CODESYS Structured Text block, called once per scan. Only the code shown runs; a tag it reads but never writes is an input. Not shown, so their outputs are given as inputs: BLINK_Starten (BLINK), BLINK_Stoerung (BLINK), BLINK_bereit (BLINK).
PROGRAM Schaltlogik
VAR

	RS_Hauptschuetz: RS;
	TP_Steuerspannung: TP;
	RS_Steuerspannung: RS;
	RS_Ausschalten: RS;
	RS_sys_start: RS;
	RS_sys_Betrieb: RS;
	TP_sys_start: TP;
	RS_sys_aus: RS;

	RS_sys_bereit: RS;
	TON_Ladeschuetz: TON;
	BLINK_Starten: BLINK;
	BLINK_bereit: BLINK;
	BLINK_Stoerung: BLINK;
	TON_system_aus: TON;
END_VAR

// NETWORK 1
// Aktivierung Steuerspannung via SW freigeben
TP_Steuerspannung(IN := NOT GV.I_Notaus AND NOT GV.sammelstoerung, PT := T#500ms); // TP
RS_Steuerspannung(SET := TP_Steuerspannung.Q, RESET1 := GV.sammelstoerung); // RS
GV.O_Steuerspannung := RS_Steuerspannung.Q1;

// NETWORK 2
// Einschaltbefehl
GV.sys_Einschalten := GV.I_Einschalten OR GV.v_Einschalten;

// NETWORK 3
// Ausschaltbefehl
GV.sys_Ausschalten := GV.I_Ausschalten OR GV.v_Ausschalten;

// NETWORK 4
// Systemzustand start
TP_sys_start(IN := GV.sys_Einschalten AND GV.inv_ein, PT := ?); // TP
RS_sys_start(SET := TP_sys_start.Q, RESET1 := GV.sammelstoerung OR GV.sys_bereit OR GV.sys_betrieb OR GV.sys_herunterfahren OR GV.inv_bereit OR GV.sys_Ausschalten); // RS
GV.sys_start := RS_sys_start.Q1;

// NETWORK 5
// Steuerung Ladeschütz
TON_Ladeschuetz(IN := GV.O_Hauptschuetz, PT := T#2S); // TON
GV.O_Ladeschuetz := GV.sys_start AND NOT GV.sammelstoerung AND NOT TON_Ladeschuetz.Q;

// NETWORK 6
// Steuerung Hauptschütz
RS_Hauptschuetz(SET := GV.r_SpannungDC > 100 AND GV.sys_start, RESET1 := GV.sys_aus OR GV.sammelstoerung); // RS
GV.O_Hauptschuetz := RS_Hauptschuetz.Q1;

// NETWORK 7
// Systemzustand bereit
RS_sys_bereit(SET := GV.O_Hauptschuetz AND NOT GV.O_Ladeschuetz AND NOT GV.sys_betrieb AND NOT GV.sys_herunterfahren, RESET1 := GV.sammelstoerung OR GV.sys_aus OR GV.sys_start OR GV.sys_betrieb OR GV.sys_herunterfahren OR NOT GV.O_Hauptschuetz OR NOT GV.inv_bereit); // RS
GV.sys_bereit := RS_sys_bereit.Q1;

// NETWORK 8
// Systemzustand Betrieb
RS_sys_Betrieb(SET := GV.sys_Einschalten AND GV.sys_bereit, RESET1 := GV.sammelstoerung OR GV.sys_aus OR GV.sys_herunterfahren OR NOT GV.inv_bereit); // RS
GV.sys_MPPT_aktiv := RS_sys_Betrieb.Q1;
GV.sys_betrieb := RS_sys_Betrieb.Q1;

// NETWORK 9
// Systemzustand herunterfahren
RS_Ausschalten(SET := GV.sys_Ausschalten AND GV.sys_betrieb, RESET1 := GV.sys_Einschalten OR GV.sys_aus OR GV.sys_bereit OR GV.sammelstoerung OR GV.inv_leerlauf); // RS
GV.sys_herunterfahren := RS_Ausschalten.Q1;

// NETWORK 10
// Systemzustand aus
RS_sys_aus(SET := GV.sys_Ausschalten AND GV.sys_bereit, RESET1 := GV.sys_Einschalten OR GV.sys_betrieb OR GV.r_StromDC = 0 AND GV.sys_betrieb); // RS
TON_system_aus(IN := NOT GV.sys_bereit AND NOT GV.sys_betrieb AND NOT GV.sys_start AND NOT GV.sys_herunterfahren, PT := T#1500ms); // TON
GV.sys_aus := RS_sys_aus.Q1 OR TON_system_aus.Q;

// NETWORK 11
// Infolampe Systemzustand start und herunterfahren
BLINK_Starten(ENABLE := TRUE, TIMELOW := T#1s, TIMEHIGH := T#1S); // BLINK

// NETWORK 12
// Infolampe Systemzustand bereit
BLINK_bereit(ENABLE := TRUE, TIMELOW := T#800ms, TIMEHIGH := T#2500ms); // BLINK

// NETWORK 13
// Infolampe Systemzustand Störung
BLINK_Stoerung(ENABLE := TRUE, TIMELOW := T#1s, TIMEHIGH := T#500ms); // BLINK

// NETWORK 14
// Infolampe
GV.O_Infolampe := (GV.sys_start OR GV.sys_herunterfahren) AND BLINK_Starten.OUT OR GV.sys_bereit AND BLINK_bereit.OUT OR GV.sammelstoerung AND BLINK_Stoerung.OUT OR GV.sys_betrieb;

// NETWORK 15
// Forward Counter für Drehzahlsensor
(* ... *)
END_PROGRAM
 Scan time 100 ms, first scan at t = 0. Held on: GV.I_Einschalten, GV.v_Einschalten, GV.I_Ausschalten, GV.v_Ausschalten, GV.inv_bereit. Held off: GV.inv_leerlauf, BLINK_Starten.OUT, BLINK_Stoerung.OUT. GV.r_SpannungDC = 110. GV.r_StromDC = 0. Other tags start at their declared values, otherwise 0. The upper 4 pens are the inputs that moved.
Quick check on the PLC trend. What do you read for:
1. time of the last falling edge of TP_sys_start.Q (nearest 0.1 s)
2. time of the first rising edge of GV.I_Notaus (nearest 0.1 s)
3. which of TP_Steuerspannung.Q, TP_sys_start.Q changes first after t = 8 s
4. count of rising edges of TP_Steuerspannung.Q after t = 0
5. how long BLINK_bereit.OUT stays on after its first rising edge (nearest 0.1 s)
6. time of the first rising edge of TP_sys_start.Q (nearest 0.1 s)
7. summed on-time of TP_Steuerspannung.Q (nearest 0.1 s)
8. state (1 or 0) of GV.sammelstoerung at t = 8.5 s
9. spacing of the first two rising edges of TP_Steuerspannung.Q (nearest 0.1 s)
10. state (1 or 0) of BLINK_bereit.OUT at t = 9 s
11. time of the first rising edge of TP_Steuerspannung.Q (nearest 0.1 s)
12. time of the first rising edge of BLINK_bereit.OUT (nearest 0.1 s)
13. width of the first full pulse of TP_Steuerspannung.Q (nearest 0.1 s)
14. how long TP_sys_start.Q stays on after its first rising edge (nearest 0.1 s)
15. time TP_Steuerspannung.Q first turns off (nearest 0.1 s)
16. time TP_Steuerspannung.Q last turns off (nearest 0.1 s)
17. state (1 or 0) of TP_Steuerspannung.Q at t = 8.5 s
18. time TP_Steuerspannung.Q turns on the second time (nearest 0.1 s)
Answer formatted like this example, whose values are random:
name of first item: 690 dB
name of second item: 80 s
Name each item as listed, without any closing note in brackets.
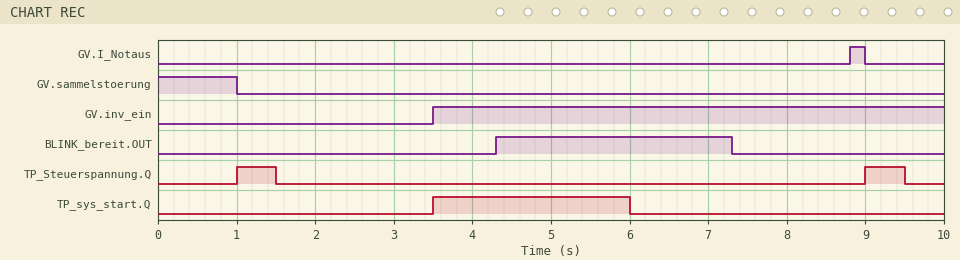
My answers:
time of the last falling edge of TP_sys_start.Q: 6.0 s
time of the first rising edge of GV.I_Notaus: 8.8 s
which of TP_Steuerspannung.Q, TP_sys_start.Q changes first after t = 8 s: TP_Steuerspannung.Q
count of rising edges of TP_Steuerspannung.Q after t = 0: 2
how long BLINK_bereit.OUT stays on after its first rising edge: 3.0 s
time of the first rising edge of TP_sys_start.Q: 3.5 s
summed on-time of TP_Steuerspannung.Q: 1.0 s
state (1 or 0) of GV.sammelstoerung at t = 8.5 s: 0
spacing of the first two rising edges of TP_Steuerspannung.Q: 8.0 s
state (1 or 0) of BLINK_bereit.OUT at t = 9 s: 0
time of the first rising edge of TP_Steuerspannung.Q: 1.0 s
time of the first rising edge of BLINK_bereit.OUT: 4.3 s
width of the first full pulse of TP_Steuerspannung.Q: 0.5 s
how long TP_sys_start.Q stays on after its first rising edge: 2.5 s
time TP_Steuerspannung.Q first turns off: 1.5 s
time TP_Steuerspannung.Q last turns off: 9.5 s
state (1 or 0) of TP_Steuerspannung.Q at t = 8.5 s: 0
time TP_Steuerspannung.Q turns on the second time: 9.0 s
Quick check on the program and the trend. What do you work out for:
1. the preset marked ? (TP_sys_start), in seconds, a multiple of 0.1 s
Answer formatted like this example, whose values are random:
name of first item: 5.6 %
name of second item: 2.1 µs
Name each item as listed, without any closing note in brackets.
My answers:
the preset marked ? (TP_sys_start), in seconds, a multiple of 0.1 s: 2.5 s
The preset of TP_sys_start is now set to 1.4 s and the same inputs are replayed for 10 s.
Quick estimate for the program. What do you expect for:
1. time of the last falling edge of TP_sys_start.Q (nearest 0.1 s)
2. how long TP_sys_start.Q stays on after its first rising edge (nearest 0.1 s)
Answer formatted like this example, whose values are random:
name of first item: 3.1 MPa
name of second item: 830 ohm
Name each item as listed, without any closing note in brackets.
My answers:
time of the last falling edge of TP_sys_start.Q: 4.9 s
how long TP_sys_start.Q stays on after its first rising edge: 1.4 s
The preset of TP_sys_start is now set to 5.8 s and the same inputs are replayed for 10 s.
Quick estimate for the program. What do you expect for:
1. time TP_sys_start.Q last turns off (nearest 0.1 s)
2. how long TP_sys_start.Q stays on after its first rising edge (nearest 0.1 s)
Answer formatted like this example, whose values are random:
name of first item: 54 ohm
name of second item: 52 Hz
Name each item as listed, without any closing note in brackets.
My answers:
time TP_sys_start.Q last turns off: 9.3 s
how long TP_sys_start.Q stays on after its first rising edge: 5.8 s
